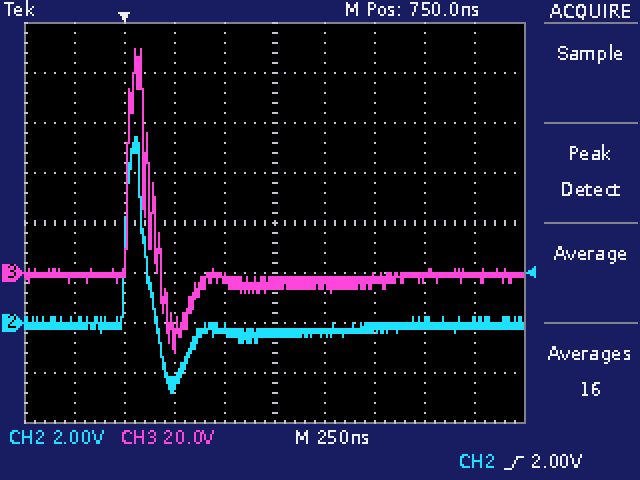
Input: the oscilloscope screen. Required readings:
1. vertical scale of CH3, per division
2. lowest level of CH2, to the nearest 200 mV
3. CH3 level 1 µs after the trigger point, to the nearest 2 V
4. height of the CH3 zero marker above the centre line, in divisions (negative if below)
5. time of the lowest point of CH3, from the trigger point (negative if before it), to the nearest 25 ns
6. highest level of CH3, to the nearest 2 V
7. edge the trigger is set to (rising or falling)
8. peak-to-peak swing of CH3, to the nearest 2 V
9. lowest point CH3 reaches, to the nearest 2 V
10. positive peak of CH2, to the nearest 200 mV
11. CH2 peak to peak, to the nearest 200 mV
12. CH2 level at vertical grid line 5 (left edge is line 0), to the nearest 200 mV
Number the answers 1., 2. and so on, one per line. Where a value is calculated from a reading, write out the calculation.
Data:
1. 20 V
2. -2.8 V
3. -4 V
4. -1.0 div
5. +250 ns
6. 90 V
7. rising
8. 90 V − (-32 V) = 122 V
9. -32 V
10. 7.4 V
11. 7.4 V − (-2.8 V) = 10.2 V
12. -400 mV
